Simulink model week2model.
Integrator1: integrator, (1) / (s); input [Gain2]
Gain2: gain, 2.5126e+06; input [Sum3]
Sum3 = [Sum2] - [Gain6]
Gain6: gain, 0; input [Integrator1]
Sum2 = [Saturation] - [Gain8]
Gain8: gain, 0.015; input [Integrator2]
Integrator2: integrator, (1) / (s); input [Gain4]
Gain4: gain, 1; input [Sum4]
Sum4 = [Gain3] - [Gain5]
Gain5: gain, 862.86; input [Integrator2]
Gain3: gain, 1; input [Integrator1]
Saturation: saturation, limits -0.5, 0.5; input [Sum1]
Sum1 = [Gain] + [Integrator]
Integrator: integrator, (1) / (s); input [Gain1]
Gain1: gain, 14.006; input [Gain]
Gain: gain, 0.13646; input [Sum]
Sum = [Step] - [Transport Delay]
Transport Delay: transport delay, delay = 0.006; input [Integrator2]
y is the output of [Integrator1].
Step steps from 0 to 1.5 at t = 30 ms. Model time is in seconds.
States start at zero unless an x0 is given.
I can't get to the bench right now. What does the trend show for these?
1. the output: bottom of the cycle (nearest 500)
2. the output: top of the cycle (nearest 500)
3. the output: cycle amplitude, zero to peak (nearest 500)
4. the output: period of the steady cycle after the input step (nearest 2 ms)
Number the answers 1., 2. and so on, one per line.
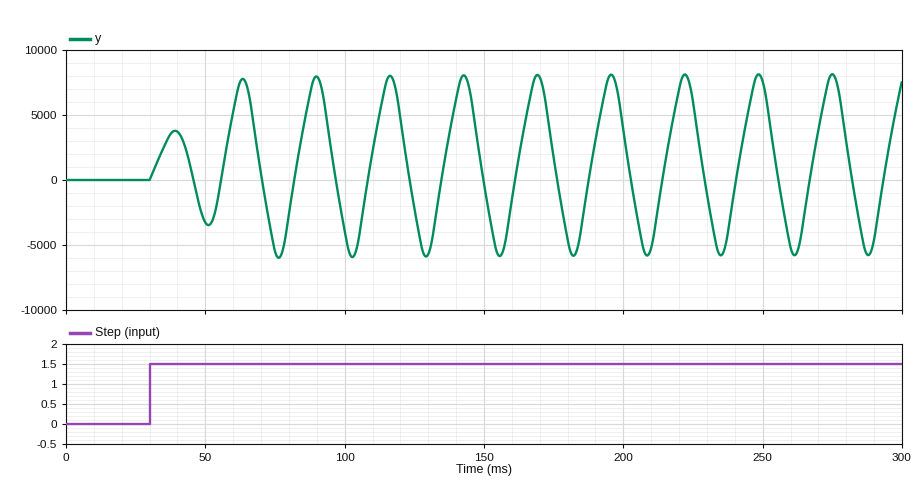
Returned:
1. -6000
2. 8000
3. 7000
4. 26 ms
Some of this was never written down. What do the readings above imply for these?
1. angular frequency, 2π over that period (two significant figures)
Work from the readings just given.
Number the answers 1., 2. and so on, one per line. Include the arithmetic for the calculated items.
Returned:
1. 2π / 26 = 0.24 rad/ms
